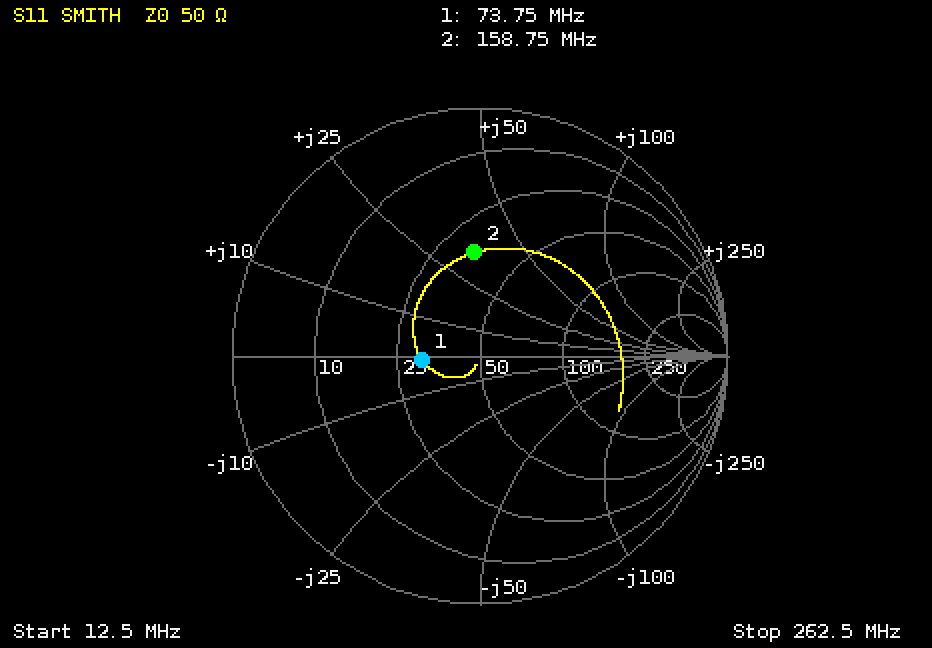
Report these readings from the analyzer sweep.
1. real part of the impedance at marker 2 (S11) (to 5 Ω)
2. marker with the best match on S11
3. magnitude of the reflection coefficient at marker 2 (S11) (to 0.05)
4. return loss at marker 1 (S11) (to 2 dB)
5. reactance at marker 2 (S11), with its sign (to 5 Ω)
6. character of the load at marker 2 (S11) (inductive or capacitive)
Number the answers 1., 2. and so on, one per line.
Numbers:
1. 35 Ω
2. marker 1
3. 0.40
4. 12 dB
5. +35 Ω
6. inductive
